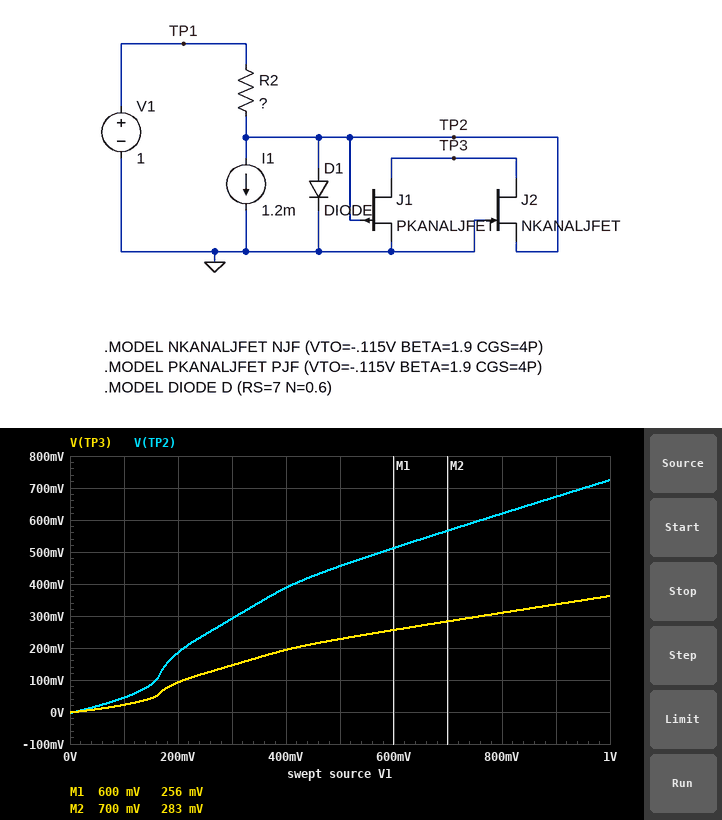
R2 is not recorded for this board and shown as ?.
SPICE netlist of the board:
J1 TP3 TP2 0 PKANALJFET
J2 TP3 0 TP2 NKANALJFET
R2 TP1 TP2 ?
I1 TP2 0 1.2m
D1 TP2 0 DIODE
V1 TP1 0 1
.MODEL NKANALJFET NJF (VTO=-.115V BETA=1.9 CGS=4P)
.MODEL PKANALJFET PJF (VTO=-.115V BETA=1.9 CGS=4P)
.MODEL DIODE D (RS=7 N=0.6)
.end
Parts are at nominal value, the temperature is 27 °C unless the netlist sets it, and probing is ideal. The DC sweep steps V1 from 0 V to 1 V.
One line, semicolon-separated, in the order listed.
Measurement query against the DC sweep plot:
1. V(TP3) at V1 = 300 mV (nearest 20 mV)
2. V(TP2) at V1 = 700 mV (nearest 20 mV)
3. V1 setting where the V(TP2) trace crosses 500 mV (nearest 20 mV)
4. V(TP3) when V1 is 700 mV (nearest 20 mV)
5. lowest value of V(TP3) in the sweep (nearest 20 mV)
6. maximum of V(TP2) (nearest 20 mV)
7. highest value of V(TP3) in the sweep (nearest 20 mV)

140 mV; 560 mV; 580 mV; 280 mV; 0 V; 720 mV; 360 mV
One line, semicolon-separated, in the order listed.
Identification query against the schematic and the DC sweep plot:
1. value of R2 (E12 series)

6.8 Ω
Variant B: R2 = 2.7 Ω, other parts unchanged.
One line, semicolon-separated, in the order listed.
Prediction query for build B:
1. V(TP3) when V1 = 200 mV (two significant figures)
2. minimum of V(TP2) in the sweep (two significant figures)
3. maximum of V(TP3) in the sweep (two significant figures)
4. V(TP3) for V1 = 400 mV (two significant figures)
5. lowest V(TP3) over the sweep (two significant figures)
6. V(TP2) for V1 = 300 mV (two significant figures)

98 mV; -2.0 mV; 420 mV; 200 mV; -1.0 mV; 300 mV
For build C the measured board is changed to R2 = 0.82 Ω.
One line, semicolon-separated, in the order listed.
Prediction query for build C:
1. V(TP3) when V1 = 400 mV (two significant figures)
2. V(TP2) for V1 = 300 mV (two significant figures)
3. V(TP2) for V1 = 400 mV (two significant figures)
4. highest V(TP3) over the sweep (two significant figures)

200 mV; 300 mV; 400 mV; 470 mV
